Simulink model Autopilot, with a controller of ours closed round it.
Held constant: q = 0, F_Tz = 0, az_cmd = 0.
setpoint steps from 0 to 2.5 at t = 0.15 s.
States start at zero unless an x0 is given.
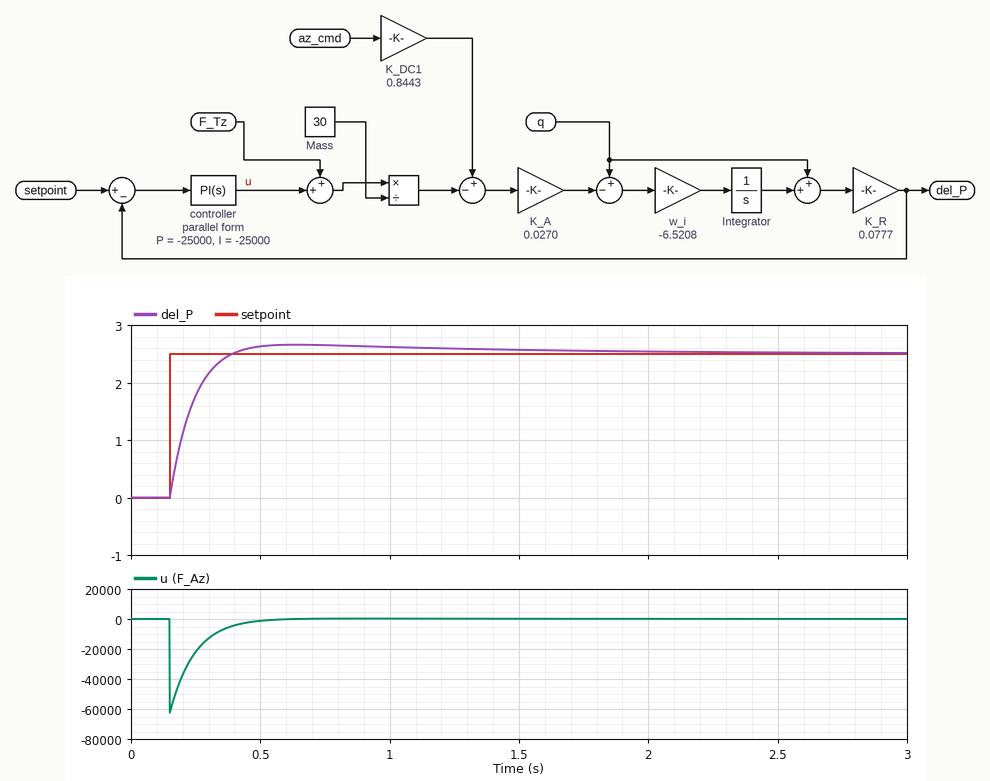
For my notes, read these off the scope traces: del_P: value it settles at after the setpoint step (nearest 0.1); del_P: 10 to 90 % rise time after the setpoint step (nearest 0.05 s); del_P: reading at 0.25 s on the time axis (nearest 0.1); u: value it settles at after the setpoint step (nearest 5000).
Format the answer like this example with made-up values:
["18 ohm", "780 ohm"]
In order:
["2.5", "0.15 s", "1.8", "0"]
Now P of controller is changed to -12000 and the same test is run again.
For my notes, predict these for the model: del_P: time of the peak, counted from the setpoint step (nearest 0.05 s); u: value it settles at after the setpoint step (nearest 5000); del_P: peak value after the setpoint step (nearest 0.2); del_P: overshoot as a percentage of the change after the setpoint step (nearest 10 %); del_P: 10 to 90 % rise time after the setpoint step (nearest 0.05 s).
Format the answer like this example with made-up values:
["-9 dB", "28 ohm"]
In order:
["0.65 s", "0", "3.0", "20 %", "0.25 s"]
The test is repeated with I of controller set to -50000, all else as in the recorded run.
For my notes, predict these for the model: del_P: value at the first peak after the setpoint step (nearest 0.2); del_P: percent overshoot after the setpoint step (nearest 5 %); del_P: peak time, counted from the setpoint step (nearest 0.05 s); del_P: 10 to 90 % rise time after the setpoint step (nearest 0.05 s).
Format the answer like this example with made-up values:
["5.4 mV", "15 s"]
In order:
["2.8", "10 %", "0.40 s", "0.15 s"]
